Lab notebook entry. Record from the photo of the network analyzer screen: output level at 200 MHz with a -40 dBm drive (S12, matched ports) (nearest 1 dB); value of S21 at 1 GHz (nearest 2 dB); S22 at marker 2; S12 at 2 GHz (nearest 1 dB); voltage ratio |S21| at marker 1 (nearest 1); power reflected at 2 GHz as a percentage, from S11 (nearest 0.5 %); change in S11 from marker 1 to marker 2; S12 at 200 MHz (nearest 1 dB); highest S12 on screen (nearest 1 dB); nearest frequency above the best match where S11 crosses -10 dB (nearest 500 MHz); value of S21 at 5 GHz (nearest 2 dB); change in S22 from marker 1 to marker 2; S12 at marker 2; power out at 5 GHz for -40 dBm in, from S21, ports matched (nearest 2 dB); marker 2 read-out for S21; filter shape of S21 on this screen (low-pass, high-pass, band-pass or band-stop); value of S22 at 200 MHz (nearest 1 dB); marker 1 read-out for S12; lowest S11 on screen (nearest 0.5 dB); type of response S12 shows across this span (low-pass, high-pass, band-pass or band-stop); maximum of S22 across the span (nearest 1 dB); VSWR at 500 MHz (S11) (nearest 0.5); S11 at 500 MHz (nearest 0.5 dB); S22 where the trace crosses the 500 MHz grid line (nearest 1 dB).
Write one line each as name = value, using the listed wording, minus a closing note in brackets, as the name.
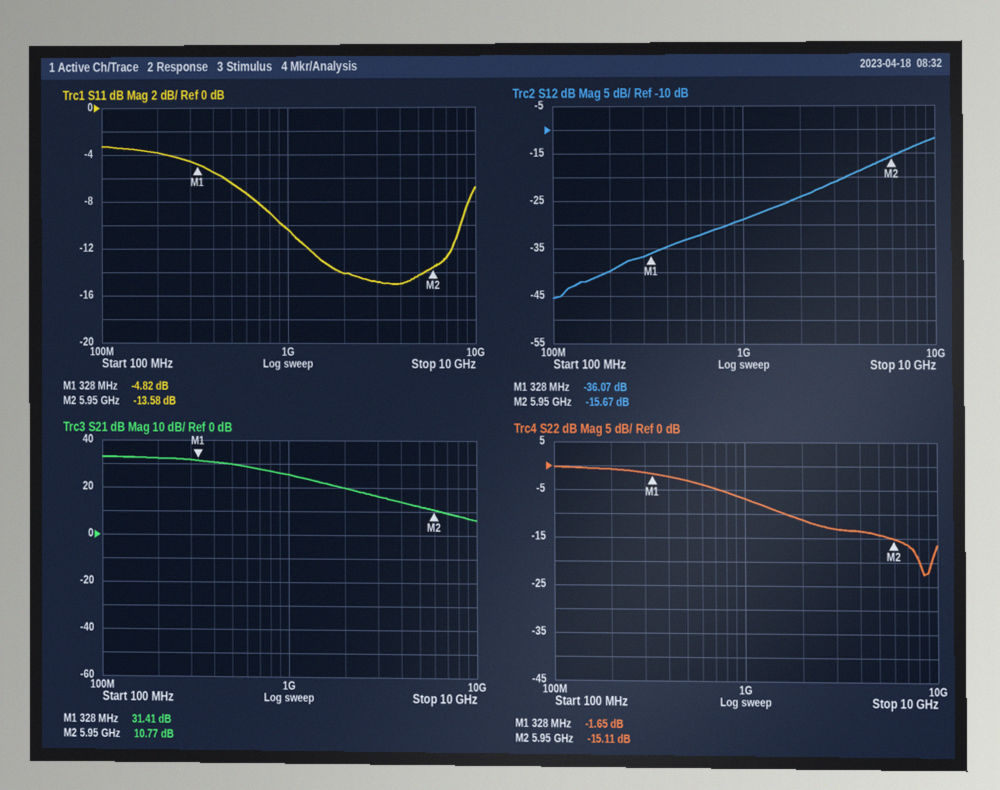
output level at 200 MHz with a -40 dBm drive (S12, matched ports) = -80 dBm
value of S21 at 1 GHz = 26 dB
S22 at marker 2 = -15.11 dB
S12 at 2 GHz = -24 dB
voltage ratio |S21| at marker 1 = 37
power reflected at 2 GHz as a percentage, from S11 = 4.0 %
change in S11 from marker 1 to marker 2 = -8.76 dB
S12 at 200 MHz = -40 dB
highest S12 on screen = -12 dB
nearest frequency above the best match where S11 crosses -10 dB = 8.5 GHz
value of S21 at 5 GHz = 12 dB
change in S22 from marker 1 to marker 2 = -13.46 dB
S12 at marker 2 = -15.67 dB
power out at 5 GHz for -40 dBm in, from S21, ports matched = -28 dBm
marker 2 read-out for S21 = 10.77 dB
filter shape of S21 on this screen = low-pass
value of S22 at 200 MHz = -1 dB
marker 1 read-out for S12 = -36.07 dB
lowest S11 on screen = -15.0 dB
type of response S12 shows across this span = high-pass
maximum of S22 across the span = 0 dB
VSWR at 500 MHz (S11) = 3.0
S11 at 500 MHz = -6.5 dB
S22 where the trace crosses the 500 MHz grid line = -3 dB
